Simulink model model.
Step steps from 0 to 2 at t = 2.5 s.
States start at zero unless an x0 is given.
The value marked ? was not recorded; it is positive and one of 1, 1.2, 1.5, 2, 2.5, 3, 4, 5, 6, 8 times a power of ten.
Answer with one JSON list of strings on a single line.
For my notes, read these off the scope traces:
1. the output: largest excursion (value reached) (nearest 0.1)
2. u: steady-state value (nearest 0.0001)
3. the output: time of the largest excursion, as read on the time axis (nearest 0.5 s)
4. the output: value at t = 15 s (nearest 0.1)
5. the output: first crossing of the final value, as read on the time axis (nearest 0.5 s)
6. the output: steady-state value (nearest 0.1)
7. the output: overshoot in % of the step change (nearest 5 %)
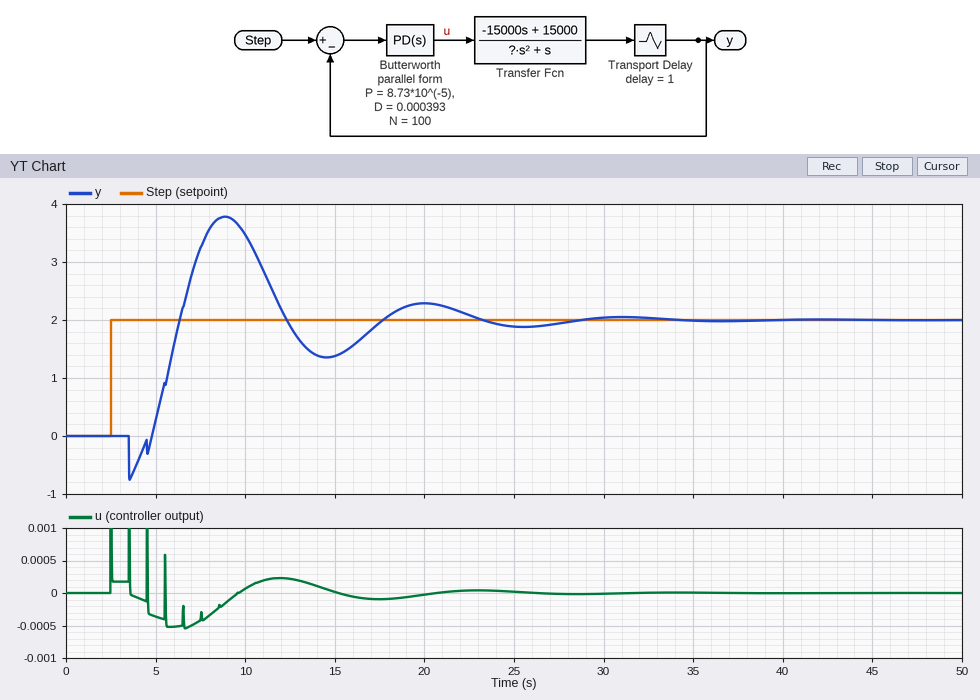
["3.8", "0.0000", "9.0 s", "1.4", "6.5 s", "2.0", "90 %"]
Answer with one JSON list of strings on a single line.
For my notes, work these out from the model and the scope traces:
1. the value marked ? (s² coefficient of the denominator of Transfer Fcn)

["15"]
